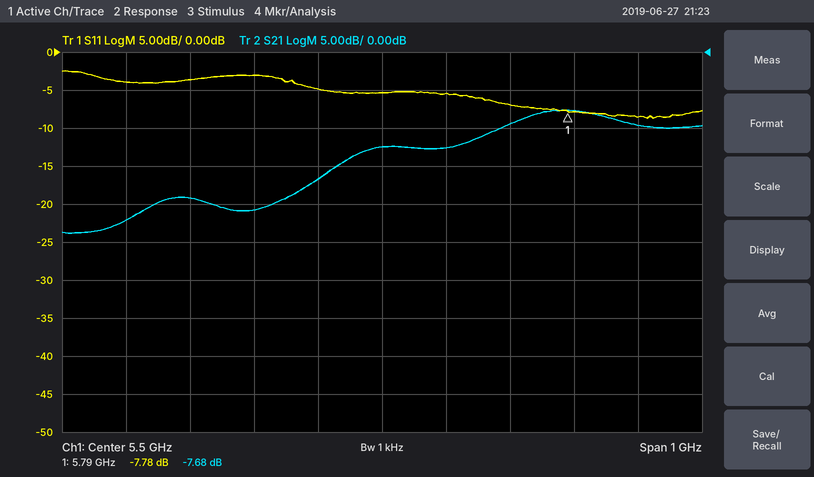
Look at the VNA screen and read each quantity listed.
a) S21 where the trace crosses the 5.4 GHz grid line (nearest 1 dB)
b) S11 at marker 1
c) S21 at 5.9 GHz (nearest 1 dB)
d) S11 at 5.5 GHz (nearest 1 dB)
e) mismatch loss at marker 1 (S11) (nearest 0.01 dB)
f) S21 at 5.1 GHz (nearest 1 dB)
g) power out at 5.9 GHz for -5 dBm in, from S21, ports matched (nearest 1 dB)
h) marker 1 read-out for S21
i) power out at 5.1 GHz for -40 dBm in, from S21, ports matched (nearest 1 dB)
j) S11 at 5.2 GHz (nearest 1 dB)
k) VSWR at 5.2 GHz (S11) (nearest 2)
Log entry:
-17 dB
-7.78 dB
-10 dB
-5 dB
0.79 dB
-22 dB
-15 dBm
-7.68 dB
-62 dBm
-4 dB
4
